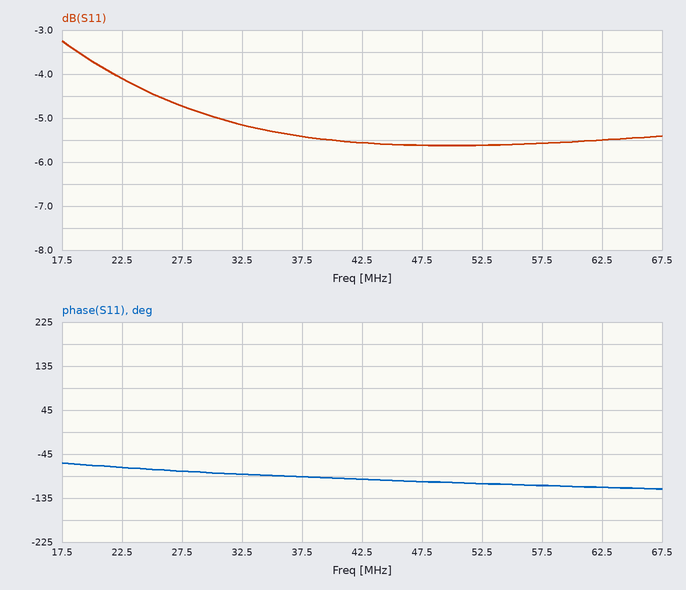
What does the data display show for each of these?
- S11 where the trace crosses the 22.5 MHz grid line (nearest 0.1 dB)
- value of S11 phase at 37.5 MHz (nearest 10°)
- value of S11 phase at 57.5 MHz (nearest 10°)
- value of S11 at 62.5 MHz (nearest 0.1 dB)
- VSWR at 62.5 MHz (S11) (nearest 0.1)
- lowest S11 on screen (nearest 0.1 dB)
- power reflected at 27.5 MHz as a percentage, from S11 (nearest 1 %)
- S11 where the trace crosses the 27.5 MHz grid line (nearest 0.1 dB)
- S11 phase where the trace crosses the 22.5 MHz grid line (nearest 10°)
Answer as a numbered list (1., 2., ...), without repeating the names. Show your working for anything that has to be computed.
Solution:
1. -4.1 dB
2. -90°
3. -110°
4. -5.5 dB
5. |Γ| = 10^(-5.5/20) = 0.5309; VSWR = (1 + 0.5309)/(1 − 0.5309) ≈ 3.3
6. -5.6 dB
7. 10^(-4.7/10) ≈ 34 %
8. -4.7 dB
9. -70°
